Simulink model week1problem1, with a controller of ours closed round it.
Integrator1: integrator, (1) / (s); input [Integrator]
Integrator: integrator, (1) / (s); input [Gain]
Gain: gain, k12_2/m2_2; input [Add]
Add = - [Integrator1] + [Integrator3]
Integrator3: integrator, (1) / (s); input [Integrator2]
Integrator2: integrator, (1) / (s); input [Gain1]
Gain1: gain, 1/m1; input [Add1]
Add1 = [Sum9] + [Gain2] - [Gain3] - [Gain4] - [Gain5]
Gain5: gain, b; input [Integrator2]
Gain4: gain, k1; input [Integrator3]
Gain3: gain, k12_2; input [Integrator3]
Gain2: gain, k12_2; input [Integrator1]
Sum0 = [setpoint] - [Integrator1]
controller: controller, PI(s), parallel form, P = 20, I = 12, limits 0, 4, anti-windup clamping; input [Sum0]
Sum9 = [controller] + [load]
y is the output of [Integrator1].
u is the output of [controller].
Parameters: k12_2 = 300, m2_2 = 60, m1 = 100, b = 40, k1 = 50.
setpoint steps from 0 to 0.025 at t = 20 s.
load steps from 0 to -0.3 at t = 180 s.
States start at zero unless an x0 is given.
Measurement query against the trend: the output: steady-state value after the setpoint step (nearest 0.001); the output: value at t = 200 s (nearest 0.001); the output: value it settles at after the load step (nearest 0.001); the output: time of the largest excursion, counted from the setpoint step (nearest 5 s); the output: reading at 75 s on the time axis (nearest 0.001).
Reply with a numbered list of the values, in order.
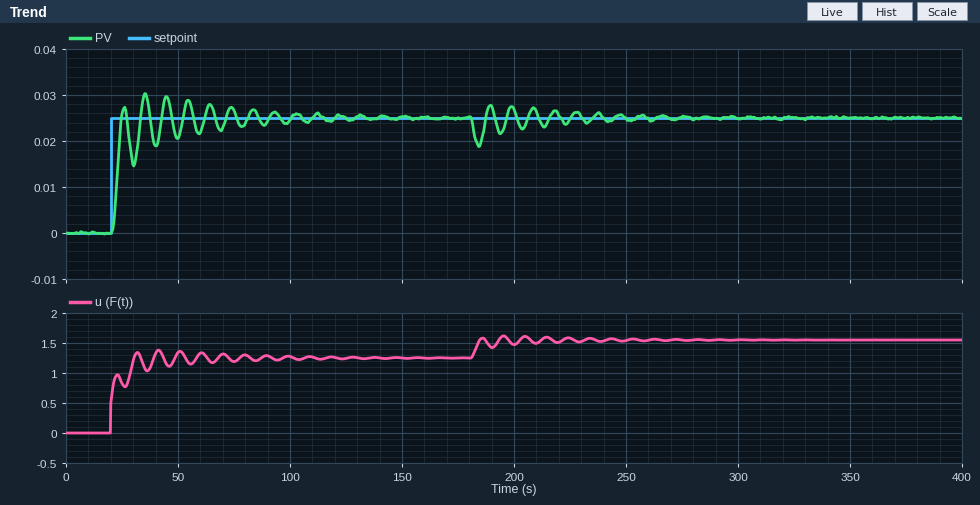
1. 0.025
2. 0.027
3. 0.025
4. 15 s
5. 0.027
